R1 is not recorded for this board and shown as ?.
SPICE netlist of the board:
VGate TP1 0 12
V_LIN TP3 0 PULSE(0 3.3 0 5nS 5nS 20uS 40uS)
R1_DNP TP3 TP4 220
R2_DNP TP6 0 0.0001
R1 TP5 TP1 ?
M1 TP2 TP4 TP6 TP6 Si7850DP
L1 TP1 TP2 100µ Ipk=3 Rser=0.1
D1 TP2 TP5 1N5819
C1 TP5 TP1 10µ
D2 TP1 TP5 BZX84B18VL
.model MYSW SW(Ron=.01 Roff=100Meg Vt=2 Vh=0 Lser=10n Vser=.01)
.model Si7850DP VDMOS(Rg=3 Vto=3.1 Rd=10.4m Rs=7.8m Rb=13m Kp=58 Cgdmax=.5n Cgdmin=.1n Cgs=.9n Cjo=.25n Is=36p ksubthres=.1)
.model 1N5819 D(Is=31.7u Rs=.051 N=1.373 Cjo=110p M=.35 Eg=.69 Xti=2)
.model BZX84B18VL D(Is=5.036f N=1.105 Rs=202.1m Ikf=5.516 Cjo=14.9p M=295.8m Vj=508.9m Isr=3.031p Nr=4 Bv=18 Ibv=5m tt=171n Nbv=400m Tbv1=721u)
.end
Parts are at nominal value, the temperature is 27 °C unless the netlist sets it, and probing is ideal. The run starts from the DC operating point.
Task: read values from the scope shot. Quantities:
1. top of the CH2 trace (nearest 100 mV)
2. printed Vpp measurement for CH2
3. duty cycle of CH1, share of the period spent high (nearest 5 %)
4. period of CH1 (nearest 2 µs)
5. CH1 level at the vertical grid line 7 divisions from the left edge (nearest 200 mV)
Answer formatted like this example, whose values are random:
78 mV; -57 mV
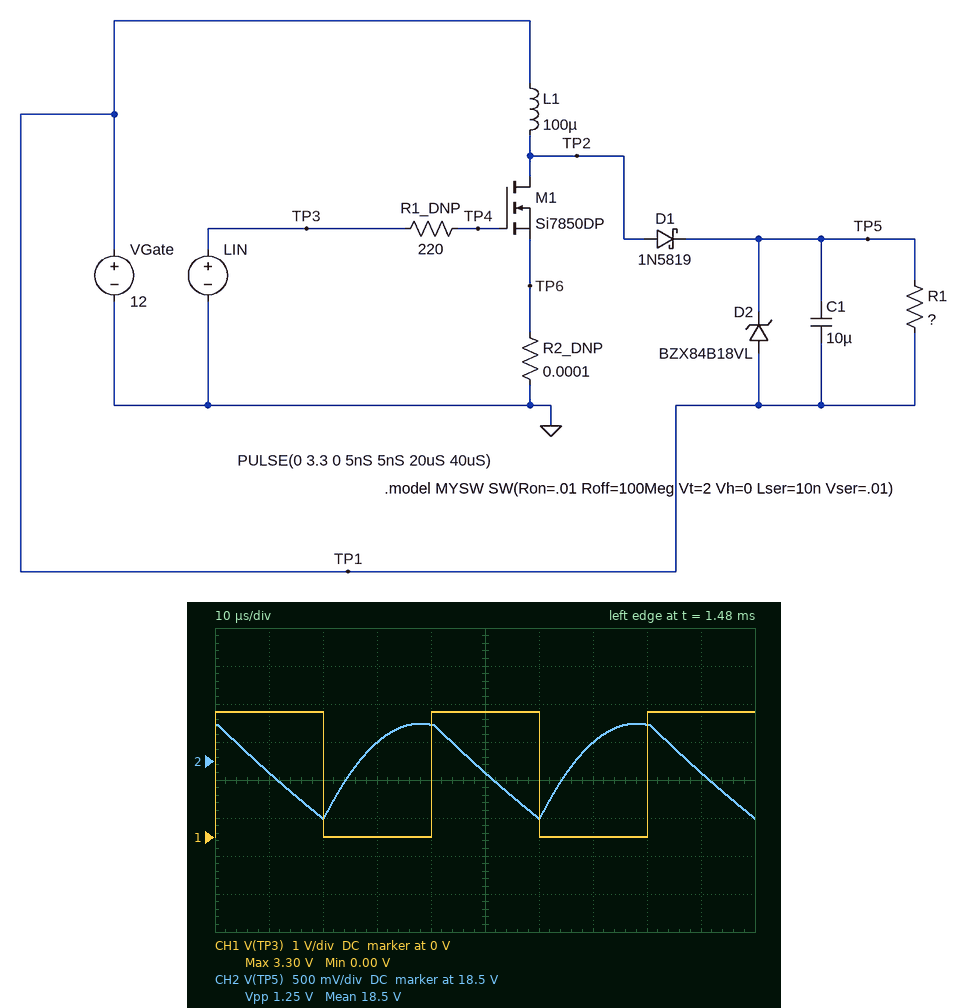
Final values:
19.0 V; 1.25 V; 50 %; 40 µs; 0 V
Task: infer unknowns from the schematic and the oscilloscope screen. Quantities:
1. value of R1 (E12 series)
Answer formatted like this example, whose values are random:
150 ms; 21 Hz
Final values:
10 Ω
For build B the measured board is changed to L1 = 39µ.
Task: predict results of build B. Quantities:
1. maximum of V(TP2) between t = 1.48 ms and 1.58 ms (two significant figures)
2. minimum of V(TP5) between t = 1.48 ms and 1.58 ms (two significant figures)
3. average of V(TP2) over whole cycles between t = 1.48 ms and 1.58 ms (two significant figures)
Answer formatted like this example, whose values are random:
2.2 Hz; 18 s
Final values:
17 V; 16 V; 12 V
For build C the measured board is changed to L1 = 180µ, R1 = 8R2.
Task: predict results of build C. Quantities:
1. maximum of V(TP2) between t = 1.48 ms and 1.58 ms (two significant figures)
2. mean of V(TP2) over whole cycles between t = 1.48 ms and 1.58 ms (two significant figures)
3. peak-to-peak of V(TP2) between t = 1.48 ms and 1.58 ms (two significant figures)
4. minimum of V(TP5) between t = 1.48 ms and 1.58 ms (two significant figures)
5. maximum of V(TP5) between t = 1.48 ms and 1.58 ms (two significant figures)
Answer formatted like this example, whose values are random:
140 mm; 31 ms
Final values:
18 V; 12 V; 15 V; 16 V; 17 V
